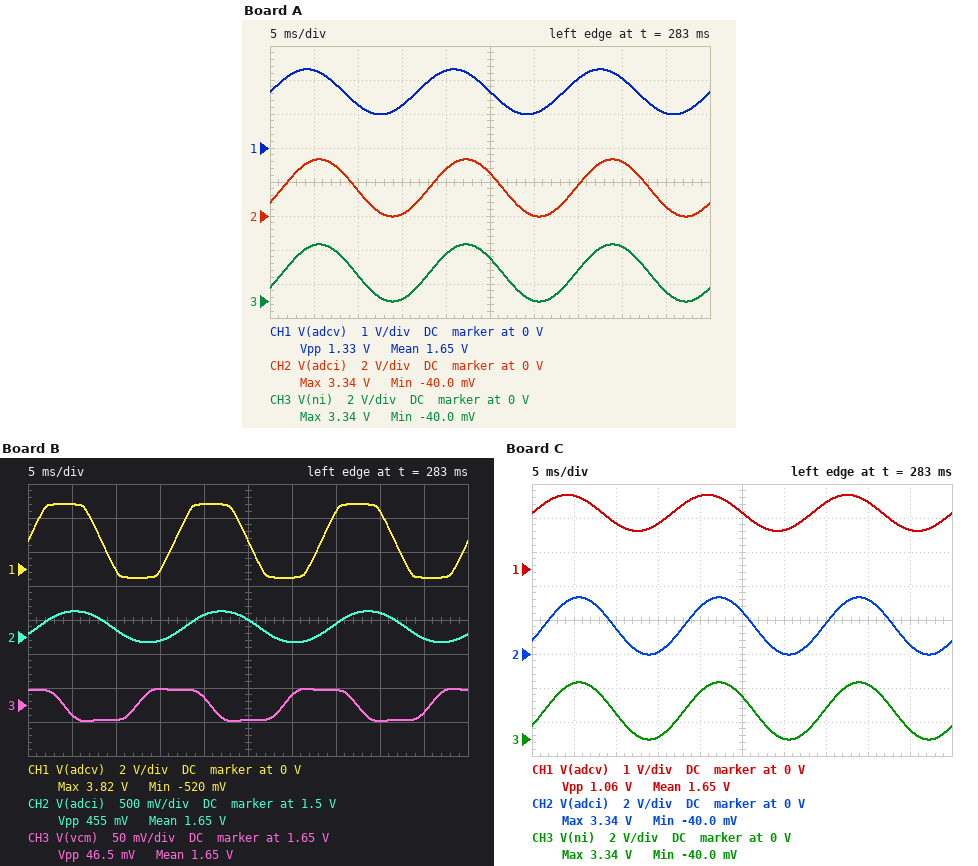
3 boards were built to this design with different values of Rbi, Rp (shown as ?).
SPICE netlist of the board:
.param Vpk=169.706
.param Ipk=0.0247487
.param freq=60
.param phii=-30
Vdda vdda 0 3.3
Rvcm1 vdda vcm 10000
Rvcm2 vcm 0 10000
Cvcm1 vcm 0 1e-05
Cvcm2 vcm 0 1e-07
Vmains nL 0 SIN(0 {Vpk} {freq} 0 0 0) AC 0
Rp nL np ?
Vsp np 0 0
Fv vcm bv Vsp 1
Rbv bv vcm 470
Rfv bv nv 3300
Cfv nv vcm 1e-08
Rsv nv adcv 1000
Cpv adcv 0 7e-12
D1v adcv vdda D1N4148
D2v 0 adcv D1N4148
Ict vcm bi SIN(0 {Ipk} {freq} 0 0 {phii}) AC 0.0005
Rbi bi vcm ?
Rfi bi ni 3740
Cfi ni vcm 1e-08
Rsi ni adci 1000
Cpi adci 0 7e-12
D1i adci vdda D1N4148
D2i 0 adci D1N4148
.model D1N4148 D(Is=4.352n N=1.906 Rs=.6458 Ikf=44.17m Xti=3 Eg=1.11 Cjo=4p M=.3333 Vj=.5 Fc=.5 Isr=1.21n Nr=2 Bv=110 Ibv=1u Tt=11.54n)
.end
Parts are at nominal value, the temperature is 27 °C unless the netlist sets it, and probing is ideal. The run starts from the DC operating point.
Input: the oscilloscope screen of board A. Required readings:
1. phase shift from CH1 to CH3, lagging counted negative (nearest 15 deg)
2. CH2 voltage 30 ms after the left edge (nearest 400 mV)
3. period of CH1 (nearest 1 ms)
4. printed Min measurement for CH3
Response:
-30 deg
0 V
17 ms
-40.0 mV
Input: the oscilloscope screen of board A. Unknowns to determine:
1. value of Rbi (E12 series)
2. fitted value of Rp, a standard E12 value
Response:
68 Ω
120 kΩ
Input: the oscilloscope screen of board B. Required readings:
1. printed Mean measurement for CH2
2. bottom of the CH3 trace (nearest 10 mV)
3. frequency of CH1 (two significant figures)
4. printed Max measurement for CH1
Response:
1.65 V
1.63 V
60 Hz
3.82 V
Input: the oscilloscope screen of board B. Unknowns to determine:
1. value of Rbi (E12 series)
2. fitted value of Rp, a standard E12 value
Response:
10 Ω
27 kΩ
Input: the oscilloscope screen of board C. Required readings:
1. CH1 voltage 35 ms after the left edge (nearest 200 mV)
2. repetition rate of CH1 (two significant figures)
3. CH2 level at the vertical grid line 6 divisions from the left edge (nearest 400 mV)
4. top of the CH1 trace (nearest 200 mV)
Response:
2.0 V
60 Hz
0 V
2.2 V
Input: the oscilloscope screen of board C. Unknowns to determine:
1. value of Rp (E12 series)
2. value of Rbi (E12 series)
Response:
150 kΩ
68 Ω
